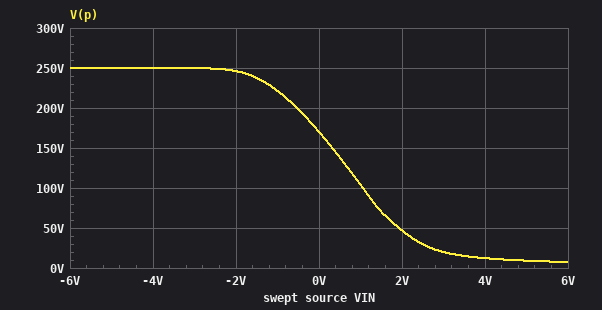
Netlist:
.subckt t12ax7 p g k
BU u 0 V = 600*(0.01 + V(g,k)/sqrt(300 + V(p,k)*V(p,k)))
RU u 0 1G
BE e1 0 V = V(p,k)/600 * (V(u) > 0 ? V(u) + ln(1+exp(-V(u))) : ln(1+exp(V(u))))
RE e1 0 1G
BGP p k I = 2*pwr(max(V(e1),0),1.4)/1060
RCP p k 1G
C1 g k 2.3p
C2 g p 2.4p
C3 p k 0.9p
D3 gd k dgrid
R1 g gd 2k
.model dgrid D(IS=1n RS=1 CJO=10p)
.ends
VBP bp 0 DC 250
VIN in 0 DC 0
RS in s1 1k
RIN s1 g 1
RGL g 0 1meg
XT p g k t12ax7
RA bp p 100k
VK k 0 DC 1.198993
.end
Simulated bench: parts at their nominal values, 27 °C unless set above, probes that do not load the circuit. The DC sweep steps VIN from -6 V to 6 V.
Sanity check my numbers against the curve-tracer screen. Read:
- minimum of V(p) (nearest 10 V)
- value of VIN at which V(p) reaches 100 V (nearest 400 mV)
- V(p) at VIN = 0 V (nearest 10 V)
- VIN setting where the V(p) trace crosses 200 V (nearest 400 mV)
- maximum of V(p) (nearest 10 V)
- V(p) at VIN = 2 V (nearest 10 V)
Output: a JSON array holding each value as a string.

["10 V", "1.2 V", "170 V", "-400 mV", "250 V", "50 V"]
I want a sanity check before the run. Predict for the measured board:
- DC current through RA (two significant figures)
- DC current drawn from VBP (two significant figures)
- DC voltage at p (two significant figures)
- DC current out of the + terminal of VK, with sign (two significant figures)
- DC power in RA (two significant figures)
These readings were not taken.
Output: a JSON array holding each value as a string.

["800 µA", "800 µA", "170 V", "-800 µA", "64 mW"]
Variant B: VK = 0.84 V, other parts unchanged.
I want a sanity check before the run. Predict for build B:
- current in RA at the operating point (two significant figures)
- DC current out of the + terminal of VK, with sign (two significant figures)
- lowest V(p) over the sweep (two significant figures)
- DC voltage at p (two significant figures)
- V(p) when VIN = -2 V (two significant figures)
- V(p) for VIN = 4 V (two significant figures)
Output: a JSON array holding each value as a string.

["1.0 mA", "-1.0 mA", "6.7 V", "150 V", "240 V", "11 V"]
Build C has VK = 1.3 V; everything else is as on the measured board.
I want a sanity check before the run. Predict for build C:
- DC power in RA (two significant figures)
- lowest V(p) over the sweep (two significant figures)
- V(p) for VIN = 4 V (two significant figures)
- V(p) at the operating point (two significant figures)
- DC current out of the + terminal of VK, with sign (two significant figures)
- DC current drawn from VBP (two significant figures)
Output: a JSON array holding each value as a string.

["54 mW", "7.7 V", "13 V", "180 V", "-740 µA", "740 µA"]
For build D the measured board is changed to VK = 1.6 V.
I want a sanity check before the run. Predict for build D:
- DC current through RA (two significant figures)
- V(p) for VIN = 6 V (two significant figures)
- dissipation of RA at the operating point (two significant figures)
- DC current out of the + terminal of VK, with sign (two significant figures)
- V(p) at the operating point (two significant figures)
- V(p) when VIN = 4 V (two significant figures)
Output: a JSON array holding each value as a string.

["570 µA", "8.5 V", "32 mW", "-570 µA", "190 V", "15 V"]
